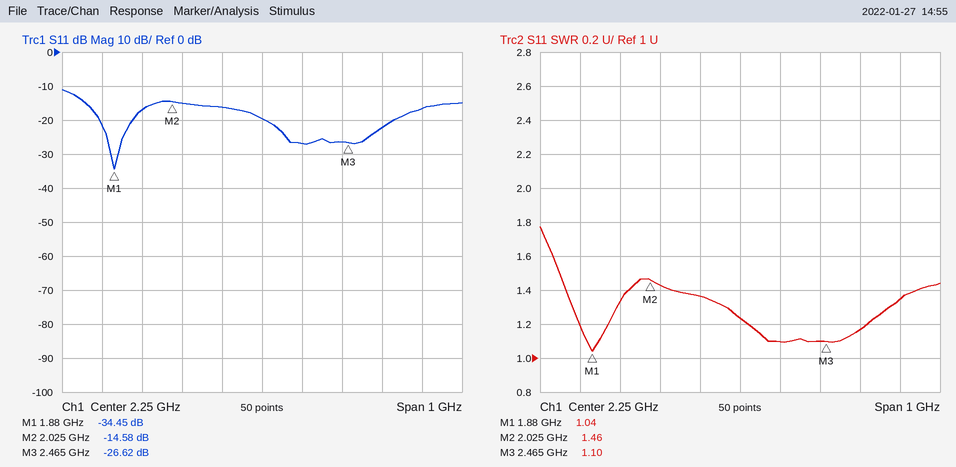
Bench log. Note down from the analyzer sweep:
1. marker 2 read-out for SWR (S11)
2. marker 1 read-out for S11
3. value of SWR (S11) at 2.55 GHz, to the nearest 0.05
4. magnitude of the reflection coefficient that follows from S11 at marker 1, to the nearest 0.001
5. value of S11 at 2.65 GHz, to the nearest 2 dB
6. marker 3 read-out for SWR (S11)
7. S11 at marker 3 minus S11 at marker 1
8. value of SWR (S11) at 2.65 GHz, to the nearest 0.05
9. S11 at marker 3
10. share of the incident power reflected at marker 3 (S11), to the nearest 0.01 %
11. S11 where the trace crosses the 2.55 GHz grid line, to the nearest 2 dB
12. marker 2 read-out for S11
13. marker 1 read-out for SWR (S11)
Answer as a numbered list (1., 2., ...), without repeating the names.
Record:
1. 1.46
2. -34.45 dB
3. 1.15
4. 0.019
5. -16 dB
6. 1.10
7. 7.83 dB
8. 1.35
9. -26.62 dB
10. 0.22 %
11. -22 dB
12. -14.58 dB
13. 1.04
